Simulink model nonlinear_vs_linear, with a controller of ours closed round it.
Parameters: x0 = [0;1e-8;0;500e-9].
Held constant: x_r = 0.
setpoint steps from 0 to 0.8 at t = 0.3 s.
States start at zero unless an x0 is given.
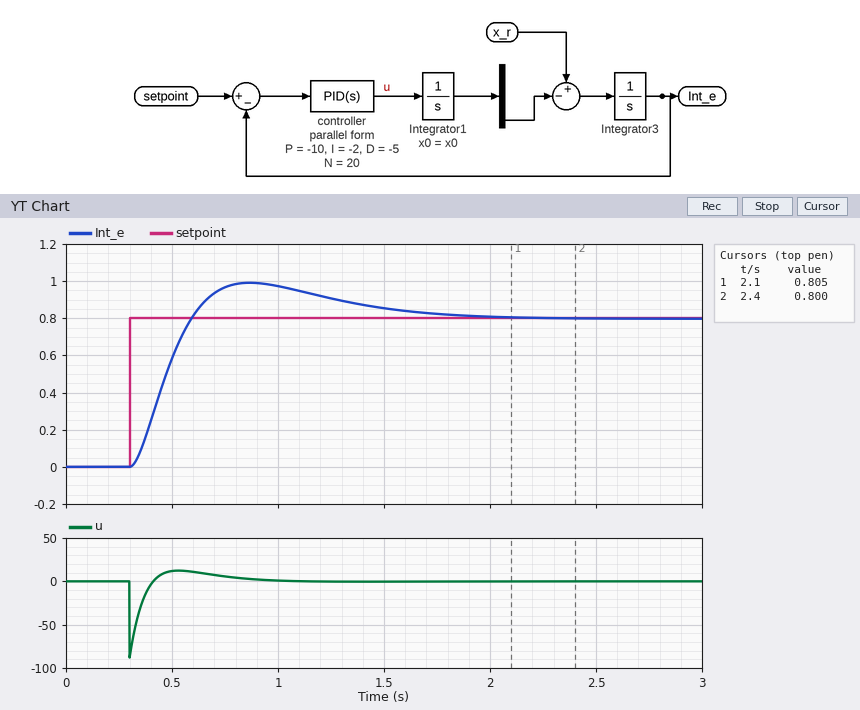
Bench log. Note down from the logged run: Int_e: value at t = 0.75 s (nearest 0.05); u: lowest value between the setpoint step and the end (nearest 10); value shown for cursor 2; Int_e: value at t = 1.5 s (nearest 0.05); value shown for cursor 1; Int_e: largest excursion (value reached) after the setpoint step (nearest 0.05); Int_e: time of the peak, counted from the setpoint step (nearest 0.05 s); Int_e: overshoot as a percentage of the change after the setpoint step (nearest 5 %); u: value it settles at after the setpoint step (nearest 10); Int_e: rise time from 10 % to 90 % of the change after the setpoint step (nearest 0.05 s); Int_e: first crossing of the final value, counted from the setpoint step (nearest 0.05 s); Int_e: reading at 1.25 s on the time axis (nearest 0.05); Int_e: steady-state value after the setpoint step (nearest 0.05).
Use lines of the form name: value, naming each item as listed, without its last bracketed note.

Int_e: value at t = 0.75 s: 0.95
u: lowest value between the setpoint step and the end: -90
value shown for cursor 2: 0.800
Int_e: value at t = 1.5 s: 0.85
value shown for cursor 1: 0.805
Int_e: largest excursion (value reached) after the setpoint step: 1.00
Int_e: time of the peak, counted from the setpoint step: 0.55 s
Int_e: overshoot as a percentage of the change after the setpoint step: 25 %
u: value it settles at after the setpoint step: 0
Int_e: rise time from 10 % to 90 % of the change after the setpoint step: 0.20 s
Int_e: first crossing of the final value, counted from the setpoint step: 0.30 s
Int_e: reading at 1.25 s on the time axis: 0.90
Int_e: steady-state value after the setpoint step: 0.80
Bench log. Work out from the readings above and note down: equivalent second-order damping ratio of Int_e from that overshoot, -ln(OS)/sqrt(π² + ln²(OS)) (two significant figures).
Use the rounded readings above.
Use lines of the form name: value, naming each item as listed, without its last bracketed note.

equivalent second-order damping ratio of Int_e from that overshoot, -ln(OS)/sqrt(π² + ln²(OS)): 0.40
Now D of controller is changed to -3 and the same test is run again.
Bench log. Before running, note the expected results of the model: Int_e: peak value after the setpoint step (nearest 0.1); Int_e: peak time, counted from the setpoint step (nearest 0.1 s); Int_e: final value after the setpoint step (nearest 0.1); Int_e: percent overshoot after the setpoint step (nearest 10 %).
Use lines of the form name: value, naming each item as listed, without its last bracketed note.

Int_e: peak value after the setpoint step: 1.1
Int_e: peak time, counted from the setpoint step: 0.7 s
Int_e: final value after the setpoint step: 0.8
Int_e: percent overshoot after the setpoint step: 40 %
